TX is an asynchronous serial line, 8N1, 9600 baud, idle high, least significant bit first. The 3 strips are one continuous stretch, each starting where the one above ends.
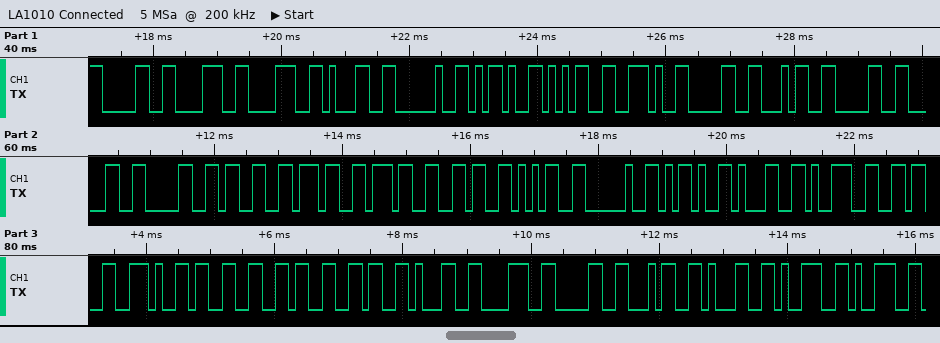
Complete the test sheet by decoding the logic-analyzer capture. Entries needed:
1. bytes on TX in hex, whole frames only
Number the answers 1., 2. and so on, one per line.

1. 30 38 38 31 20 2D 35 2E 30 34 30 30 30 33 37 37 36 35 20 2D 31 39 36 2E 33 36 36 31 38 30 34 31 39 39
